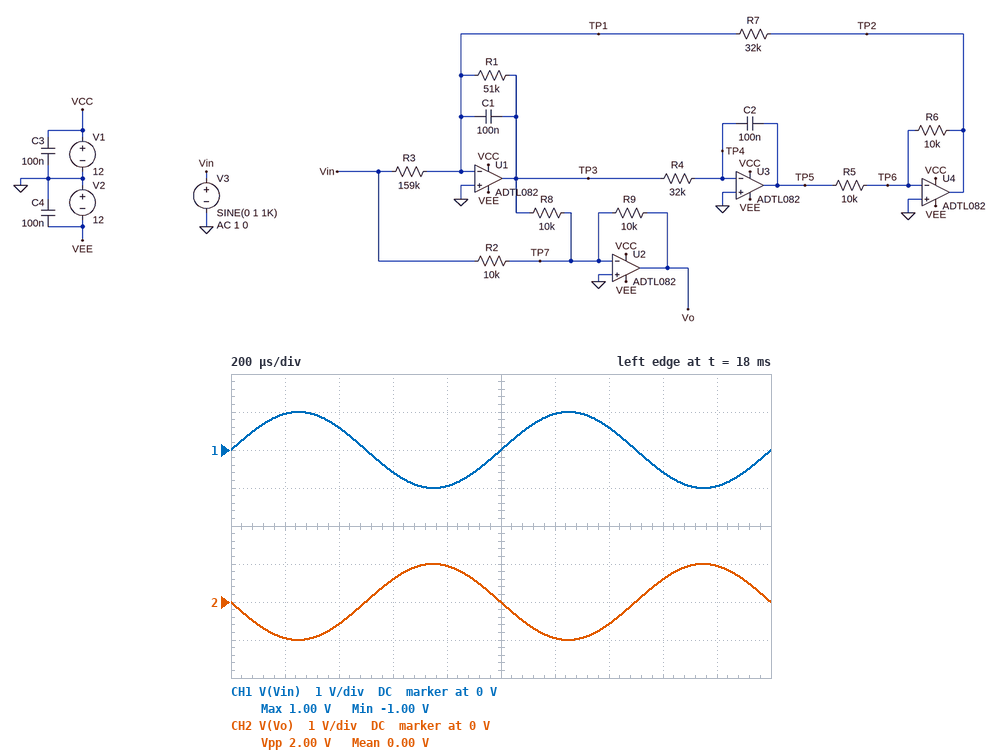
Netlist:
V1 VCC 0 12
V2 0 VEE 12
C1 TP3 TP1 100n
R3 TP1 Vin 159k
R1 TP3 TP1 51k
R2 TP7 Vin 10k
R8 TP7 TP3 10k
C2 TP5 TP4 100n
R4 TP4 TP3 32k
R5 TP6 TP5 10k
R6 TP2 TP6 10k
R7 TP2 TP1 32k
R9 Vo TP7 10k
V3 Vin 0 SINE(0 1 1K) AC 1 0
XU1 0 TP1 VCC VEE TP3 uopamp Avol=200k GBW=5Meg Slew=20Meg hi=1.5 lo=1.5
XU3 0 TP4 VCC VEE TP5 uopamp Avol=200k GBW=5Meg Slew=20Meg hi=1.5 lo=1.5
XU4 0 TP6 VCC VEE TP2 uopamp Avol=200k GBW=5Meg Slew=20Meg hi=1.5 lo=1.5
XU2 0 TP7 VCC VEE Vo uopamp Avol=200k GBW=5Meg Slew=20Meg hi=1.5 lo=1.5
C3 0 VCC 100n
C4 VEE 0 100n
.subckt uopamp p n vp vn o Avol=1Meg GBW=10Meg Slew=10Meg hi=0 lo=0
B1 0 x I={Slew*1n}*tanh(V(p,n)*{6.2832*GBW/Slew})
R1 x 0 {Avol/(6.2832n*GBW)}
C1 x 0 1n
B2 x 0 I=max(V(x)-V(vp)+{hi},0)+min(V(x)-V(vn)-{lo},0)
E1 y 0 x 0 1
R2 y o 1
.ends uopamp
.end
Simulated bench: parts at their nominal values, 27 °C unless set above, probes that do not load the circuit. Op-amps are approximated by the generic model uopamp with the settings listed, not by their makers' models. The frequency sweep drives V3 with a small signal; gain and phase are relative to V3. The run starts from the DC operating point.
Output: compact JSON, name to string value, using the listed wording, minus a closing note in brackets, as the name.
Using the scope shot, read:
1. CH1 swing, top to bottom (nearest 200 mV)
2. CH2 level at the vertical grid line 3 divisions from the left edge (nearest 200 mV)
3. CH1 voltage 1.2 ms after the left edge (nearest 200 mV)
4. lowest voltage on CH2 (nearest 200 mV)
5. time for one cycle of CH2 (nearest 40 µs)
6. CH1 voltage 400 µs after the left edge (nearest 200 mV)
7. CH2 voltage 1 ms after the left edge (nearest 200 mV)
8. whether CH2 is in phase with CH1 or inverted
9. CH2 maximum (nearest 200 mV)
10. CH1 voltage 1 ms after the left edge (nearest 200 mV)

{"CH1 swing, top to bottom": "2.0 V", "CH2 level at the vertical grid line 3 divisions from the left edge": "600 mV", "CH1 voltage 1.2 ms after the left edge": "1.0 V", "lowest voltage on CH2": "-1.0 V", "time for one cycle of CH2": "1.00 ms", "CH1 voltage 400 µs after the left edge": "600 mV", "CH2 voltage 1 ms after the left edge": "0 V", "whether CH2 is in phase with CH1 or inverted": "inverted", "CH2 maximum": "1.0 V", "CH1 voltage 1 ms after the left edge": "0 V"}
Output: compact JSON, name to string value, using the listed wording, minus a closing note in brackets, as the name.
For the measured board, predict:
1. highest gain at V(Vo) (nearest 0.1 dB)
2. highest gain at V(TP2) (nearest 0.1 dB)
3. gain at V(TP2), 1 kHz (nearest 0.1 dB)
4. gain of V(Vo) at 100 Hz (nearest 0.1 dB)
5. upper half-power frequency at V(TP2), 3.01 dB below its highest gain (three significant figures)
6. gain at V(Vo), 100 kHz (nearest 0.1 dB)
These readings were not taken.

{"highest gain at V(Vo)": "0 dB", "highest gain at V(TP2)": "-9.4 dB", "gain at V(TP2), 1 kHz": "-66.0 dB", "gain of V(Vo) at 100 Hz": "-0.4 dB", "upper half-power frequency at V(TP2), 3.01 dB below its highest gain": "58.8 Hz", "gain at V(Vo), 100 kHz": "0 dB"}
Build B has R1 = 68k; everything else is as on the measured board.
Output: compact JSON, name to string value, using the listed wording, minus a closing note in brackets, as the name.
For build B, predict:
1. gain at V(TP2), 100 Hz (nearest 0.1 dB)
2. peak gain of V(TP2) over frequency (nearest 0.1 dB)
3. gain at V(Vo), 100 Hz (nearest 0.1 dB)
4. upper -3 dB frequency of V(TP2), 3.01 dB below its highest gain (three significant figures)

{"gain at V(TP2), 100 Hz": "-24.0 dB", "peak gain of V(TP2) over frequency": "-7.1 dB", "gain at V(Vo), 100 Hz": "-0.3 dB", "upper -3 dB frequency of V(TP2), 3.01 dB below its highest gain": "57.7 Hz"}
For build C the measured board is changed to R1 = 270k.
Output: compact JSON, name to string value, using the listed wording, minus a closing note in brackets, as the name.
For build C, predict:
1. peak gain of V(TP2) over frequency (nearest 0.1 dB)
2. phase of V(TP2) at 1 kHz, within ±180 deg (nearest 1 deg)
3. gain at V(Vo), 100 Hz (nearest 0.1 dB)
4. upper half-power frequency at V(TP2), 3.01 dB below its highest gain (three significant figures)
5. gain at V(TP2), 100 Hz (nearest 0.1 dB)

{"peak gain of V(TP2) over frequency": "4.6 dB", "phase of V(TP2) at 1 kHz, within ±180 deg": "0 deg", "gain at V(Vo), 100 Hz": "0 dB", "upper half-power frequency at V(TP2), 3.01 dB below its highest gain": "52.4 Hz", "gain at V(TP2), 100 Hz": "-23.6 dB"}
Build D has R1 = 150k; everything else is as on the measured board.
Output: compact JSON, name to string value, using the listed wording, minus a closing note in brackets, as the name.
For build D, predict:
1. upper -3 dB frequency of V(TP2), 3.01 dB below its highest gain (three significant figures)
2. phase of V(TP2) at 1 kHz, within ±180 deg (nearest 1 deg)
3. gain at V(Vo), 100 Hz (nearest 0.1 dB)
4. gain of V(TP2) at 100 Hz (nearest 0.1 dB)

{"upper -3 dB frequency of V(TP2), 3.01 dB below its highest gain": "54.2 Hz", "phase of V(TP2) at 1 kHz, within ±180 deg": "1 deg", "gain at V(Vo), 100 Hz": "-0.1 dB", "gain of V(TP2) at 100 Hz": "-23.7 dB"}
